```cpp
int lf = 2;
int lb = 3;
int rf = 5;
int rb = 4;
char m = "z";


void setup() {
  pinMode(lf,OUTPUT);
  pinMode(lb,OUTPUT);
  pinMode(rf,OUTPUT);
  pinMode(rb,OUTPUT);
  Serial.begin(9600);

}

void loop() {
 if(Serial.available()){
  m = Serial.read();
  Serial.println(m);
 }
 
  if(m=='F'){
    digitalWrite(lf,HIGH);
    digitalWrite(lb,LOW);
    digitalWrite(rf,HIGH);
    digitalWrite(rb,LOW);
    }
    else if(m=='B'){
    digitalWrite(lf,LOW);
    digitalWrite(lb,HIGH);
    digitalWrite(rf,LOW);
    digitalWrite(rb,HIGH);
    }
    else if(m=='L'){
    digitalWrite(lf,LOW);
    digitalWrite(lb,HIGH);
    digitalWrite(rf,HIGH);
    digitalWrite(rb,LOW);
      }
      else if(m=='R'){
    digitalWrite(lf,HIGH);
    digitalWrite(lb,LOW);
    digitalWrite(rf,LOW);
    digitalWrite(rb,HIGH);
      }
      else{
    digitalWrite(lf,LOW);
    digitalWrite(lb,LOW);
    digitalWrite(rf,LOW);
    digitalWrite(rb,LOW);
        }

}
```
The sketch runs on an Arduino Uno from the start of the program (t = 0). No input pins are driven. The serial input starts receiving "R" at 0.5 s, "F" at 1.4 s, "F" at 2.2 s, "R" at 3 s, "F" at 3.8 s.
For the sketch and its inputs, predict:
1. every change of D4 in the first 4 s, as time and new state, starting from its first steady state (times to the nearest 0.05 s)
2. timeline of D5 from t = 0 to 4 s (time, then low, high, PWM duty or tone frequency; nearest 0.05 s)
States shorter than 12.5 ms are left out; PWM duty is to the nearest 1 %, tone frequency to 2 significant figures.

0 s low; 0.5 s high; 1.4 s low; 3 s high; 3.8 s low
0 s low; 1.4 s high; 3 s low; 3.8 s high
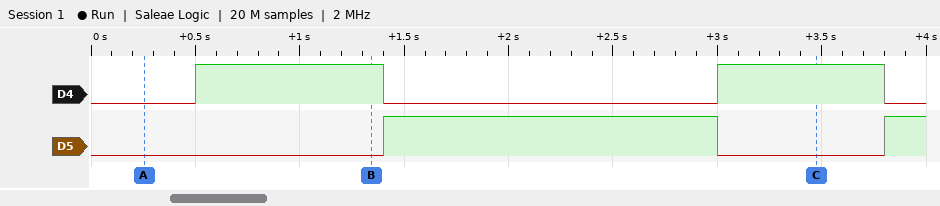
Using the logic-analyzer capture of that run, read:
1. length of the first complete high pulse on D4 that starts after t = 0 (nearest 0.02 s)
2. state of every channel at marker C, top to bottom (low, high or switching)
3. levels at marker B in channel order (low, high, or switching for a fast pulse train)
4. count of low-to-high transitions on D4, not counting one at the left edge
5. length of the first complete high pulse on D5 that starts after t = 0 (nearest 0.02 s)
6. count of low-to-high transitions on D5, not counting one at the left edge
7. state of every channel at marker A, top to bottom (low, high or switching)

0.90 s
D4 high, D5 low
D4 high, D5 low
2
1.60 s
2
D4 low, D5 low
